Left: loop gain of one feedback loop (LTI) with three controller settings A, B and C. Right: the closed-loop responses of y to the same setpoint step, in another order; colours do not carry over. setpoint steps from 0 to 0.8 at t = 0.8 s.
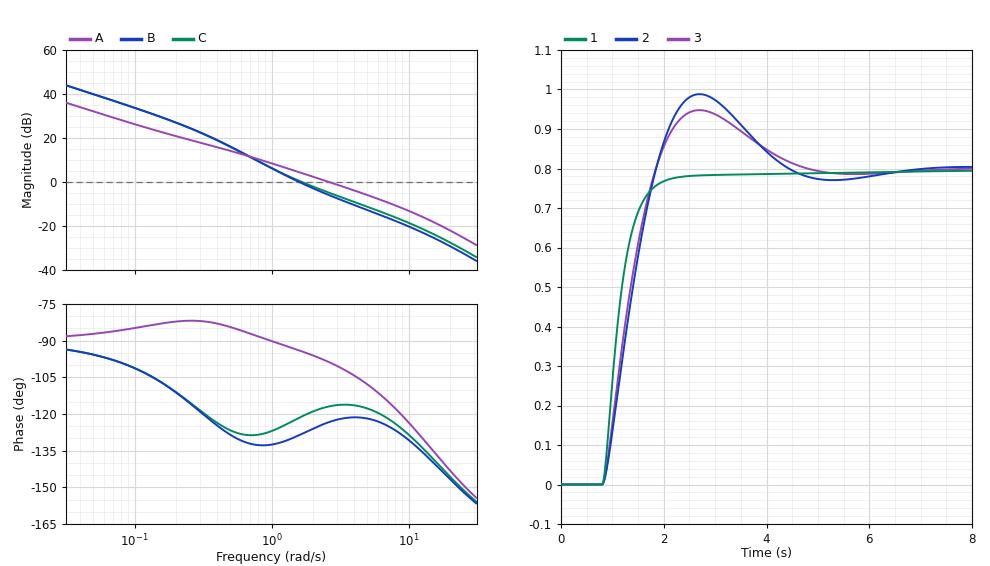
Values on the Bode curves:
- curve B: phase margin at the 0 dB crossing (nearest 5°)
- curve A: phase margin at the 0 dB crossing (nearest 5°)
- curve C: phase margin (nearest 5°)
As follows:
50°
80°
60°
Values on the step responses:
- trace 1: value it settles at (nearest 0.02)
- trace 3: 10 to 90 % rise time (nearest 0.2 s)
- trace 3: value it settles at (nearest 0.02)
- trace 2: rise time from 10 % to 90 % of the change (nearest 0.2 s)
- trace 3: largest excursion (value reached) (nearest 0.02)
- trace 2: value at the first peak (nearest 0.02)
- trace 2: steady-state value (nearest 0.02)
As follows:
0.80
0.8 s
0.80
0.8 s
0.94
0.98
0.80
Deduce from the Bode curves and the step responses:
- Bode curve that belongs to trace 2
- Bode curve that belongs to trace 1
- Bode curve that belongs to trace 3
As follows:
B
A
C
